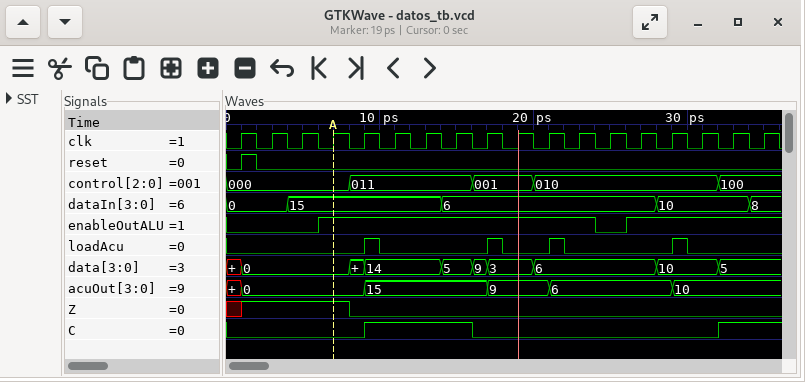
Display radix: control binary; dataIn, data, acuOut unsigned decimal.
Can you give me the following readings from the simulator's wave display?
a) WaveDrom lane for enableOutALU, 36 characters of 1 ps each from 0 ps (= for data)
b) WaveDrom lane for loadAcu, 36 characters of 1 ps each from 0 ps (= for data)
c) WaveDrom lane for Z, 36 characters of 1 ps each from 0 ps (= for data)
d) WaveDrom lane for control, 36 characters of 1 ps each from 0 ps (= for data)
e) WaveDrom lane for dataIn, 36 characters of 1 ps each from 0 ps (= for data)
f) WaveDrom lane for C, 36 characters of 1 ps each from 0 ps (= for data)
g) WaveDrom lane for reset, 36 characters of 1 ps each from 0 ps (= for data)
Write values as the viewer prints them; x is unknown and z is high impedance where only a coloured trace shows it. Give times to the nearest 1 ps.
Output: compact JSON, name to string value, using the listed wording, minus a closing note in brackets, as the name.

{"WaveDrom lane for enableOutALU, 36 characters of 1 ps each from 0 ps": "{name: 'enableOutALU', wave: '0.....1.................0.1.........'}", "WaveDrom lane for loadAcu, 36 characters of 1 ps each from 0 ps": "{name: 'loadAcu', wave: '0........10......10..10......10.....'}", "WaveDrom lane for Z, 36 characters of 1 ps each from 0 ps": "{name: 'Z', wave: 'x1......0...........................'}", "WaveDrom lane for control, 36 characters of 1 ps each from 0 ps": "{name: 'control', wave: '=.......=.......=...=...........=...', data: '000 011 001 010 100'}", "WaveDrom lane for dataIn, 36 characters of 1 ps each from 0 ps": "{name: 'dataIn', wave: '=...=.........=.............=.....=.', data: '0 15 6 10 8'}", "WaveDrom lane for C, 36 characters of 1 ps each from 0 ps": "{name: 'C', wave: '0........1......0...............1...'}", "WaveDrom lane for reset, 36 characters of 1 ps each from 0 ps": "{name: 'reset', wave: '010.................................'}"}
